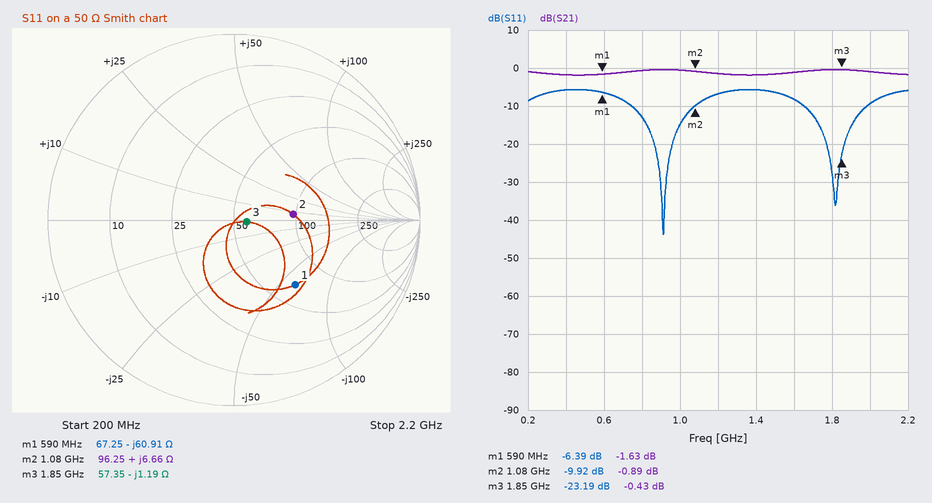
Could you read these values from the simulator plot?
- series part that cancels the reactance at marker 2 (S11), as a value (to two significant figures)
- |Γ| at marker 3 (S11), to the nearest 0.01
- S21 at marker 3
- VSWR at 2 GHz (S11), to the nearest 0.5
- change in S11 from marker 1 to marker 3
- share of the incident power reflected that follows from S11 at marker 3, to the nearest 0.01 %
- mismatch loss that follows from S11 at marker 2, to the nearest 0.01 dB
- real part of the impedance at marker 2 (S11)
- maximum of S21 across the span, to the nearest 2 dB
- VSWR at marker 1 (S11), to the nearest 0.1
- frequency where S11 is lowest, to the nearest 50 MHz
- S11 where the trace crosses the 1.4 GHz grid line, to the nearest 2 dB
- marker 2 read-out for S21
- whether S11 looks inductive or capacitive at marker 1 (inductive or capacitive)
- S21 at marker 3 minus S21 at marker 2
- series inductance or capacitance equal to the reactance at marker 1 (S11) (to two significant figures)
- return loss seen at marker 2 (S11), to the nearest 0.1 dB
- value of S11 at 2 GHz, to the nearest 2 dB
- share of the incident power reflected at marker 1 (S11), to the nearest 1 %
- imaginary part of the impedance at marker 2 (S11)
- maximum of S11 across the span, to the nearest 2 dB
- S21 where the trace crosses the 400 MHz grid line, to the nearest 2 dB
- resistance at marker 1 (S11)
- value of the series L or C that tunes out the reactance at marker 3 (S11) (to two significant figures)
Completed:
22 pF
0.07
-0.43 dB
2.0
-16.80 dB
0.48 %
0.47 dB
96.25 Ω
0 dB
2.8
900 MHz
-6 dB
-0.89 dB
capacitive
0.46 dB
4.4 pF
9.9 dB
-10 dB
23 %
+6.66 Ω
-6 dB
-2 dB
67.25 Ω
100 pH
